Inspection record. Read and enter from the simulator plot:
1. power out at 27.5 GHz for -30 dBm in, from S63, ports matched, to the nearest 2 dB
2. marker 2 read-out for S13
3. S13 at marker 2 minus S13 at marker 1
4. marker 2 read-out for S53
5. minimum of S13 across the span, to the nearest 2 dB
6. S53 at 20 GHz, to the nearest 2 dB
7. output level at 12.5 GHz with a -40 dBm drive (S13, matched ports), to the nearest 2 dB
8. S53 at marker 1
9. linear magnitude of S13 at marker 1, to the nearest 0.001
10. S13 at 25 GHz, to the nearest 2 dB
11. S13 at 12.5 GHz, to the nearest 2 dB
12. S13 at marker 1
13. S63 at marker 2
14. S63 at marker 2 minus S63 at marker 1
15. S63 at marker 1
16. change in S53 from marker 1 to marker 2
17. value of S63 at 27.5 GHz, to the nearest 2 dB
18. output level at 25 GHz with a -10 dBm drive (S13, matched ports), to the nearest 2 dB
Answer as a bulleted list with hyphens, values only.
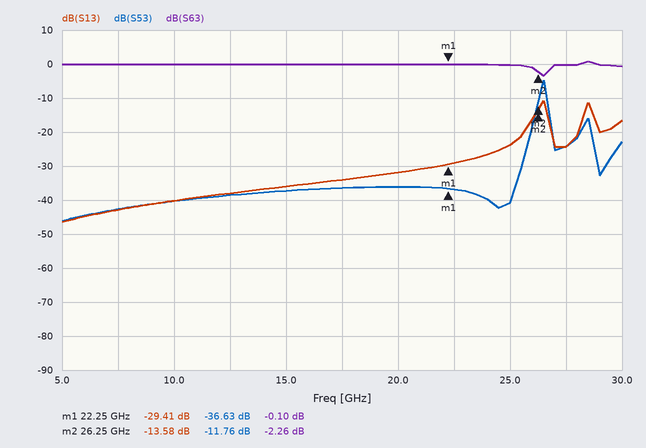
- -30 dBm
- -13.58 dB
- 15.83 dB
- -11.76 dB
- -46 dB
- -36 dB
- -78 dBm
- -36.63 dB
- 0.034
- -24 dB
- -38 dB
- -29.41 dB
- -2.26 dB
- -2.16 dB
- -0.10 dB
- 24.87 dB
- 0 dB
- -34 dBm
